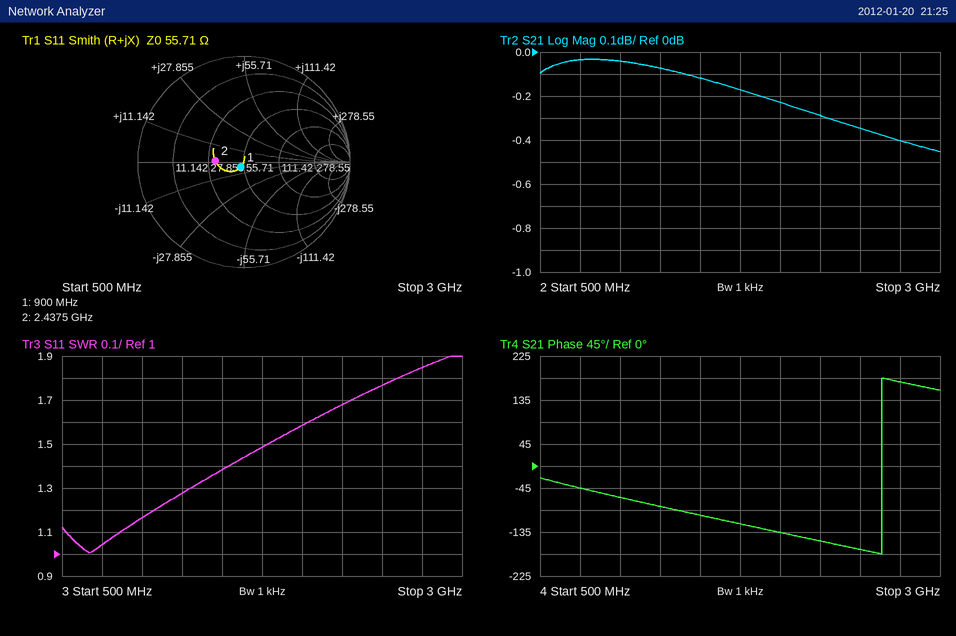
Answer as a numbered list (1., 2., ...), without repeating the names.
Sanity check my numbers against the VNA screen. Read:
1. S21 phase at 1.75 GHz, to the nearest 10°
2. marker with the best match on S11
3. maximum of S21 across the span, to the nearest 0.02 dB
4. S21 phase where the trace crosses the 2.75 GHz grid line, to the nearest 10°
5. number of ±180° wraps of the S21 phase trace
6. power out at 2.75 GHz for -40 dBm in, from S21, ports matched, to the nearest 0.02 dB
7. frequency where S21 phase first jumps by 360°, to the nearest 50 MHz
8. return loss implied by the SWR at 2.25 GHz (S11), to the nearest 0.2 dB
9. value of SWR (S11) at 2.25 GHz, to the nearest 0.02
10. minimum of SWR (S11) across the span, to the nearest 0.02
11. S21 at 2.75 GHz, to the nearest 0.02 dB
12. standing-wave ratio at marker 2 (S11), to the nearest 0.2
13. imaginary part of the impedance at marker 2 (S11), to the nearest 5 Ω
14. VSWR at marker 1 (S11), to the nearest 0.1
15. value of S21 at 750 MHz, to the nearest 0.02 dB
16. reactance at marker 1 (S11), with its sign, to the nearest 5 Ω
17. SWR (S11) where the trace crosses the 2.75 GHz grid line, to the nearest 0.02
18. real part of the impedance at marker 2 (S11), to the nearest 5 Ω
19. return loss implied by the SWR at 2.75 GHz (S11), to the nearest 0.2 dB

1. -120°
2. marker 1
3. -0.04 dB
4. 170°
5. 1
6. -40.40 dBm
7. 2.65 GHz
8. 12.0 dB
9. 1.68
10. 1.00
11. -0.40 dB
12. 1.8
13. 0 Ω
14. 1.1
15. -0.04 dB
16. -5 Ω
17. 1.84
18. 30 Ω
19. 10.6 dB
